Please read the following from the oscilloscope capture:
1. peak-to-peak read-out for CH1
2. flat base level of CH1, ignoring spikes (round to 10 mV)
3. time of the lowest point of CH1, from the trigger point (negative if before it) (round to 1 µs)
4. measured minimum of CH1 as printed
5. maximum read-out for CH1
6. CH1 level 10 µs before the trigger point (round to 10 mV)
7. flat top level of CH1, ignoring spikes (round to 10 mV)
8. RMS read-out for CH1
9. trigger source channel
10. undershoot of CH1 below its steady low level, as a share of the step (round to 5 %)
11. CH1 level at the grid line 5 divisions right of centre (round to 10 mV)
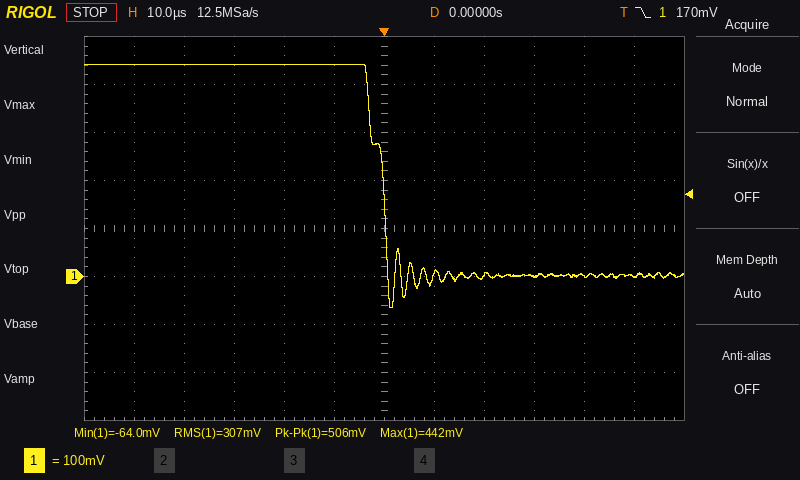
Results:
506 mV
0 mV
+1 µs
-64.0 mV
442 mV
440 mV
440 mV
307 mV
CH1
15 %
0 mV
